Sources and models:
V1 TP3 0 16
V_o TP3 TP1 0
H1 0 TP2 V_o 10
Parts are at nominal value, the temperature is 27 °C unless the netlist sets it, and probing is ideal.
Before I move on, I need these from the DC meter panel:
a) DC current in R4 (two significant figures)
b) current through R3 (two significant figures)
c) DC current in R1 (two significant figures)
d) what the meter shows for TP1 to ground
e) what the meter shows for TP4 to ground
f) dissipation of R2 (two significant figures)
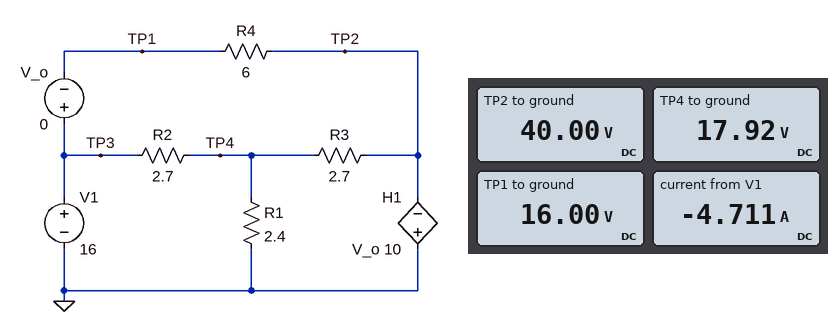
4.0 A
8.2 A
7.5 A
16.00 V
17.92 V
1.4 W
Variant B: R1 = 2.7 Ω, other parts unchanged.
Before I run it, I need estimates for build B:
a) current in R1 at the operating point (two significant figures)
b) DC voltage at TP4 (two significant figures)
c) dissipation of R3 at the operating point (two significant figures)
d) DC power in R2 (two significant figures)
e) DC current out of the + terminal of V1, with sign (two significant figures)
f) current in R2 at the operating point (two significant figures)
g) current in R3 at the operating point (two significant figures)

6.9 A
19 V
170 W
2.6 W
-5.0 A
990 mA
7.9 A
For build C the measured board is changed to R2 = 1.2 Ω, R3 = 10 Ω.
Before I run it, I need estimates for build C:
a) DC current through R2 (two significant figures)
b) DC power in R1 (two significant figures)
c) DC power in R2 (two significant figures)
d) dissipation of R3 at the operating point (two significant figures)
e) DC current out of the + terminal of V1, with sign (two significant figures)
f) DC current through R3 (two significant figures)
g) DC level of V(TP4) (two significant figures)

2.6 A
69 W
8.3 W
74 W
-1.4 A
2.7 A
13 V
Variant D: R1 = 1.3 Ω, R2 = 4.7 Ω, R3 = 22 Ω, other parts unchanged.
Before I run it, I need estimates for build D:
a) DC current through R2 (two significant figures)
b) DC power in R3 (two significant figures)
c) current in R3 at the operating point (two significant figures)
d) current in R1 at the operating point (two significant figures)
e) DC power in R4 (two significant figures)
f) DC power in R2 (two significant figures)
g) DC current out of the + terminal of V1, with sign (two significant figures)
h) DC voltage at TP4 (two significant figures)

2.3 A
55 W
1.6 A
3.9 A
96 W
25 W
-1.7 A
5.1 V
